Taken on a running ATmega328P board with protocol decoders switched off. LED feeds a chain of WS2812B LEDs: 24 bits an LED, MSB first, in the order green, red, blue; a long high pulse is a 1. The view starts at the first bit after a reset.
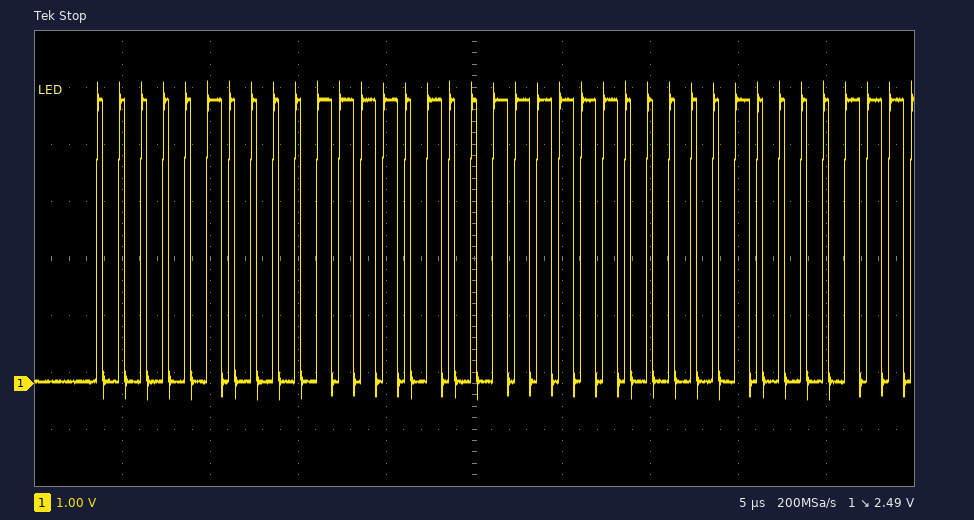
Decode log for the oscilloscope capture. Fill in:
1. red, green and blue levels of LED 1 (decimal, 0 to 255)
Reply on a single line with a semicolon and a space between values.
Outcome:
61, 4, 63
